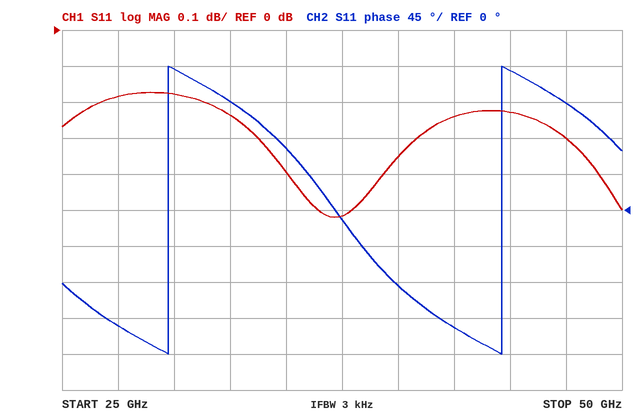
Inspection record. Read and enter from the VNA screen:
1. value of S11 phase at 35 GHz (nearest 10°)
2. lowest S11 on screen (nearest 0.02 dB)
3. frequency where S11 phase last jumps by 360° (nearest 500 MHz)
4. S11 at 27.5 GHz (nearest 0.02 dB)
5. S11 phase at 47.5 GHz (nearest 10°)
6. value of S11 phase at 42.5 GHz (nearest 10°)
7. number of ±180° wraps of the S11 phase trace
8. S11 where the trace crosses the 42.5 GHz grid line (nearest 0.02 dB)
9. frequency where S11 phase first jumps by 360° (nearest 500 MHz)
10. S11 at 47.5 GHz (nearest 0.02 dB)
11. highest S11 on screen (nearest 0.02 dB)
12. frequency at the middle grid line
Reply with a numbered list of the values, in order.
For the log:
1. 80°
2. -0.52 dB
3. 44.5 GHz
4. -0.18 dB
5. 130°
6. -150°
7. 2
8. -0.24 dB
9. 30.0 GHz
10. -0.30 dB
11. -0.18 dB
12. 37.5 GHz
